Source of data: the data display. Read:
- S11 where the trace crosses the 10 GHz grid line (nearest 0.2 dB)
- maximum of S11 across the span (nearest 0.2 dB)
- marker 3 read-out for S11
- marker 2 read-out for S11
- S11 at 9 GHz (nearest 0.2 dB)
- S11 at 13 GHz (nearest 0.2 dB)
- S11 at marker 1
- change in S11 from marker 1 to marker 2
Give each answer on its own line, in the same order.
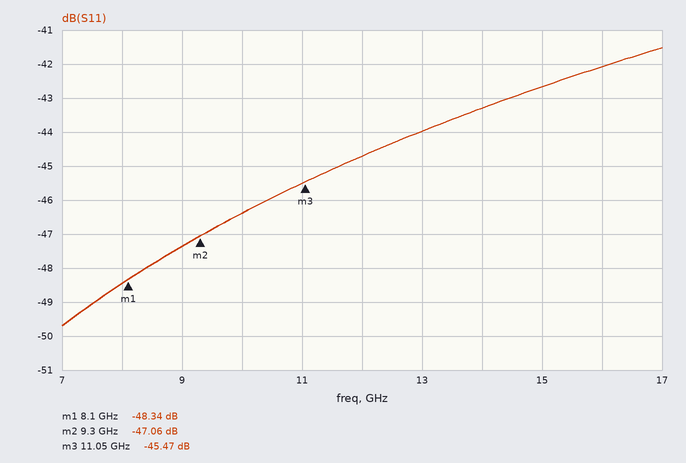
-46.4 dB
-41.6 dB
-45.47 dB
-47.06 dB
-47.4 dB
-44.0 dB
-48.34 dB
1.28 dB
